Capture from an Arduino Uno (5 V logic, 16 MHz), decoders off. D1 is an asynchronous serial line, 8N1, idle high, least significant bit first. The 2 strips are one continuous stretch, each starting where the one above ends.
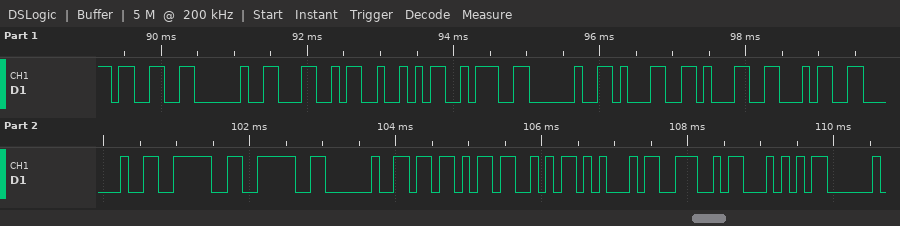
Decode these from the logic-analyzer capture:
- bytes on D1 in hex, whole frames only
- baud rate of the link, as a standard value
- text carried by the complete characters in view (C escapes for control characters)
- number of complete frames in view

0x33 0x20 0x4C 0x52 0x3A 0x20 0x31 0x31 0x34 0x20 0x3E 0x3E 0x20 0x5B 0x53 0x45 0x4E 0x54
9600 baud
"3 LR: 114 >> [SENT"
18
